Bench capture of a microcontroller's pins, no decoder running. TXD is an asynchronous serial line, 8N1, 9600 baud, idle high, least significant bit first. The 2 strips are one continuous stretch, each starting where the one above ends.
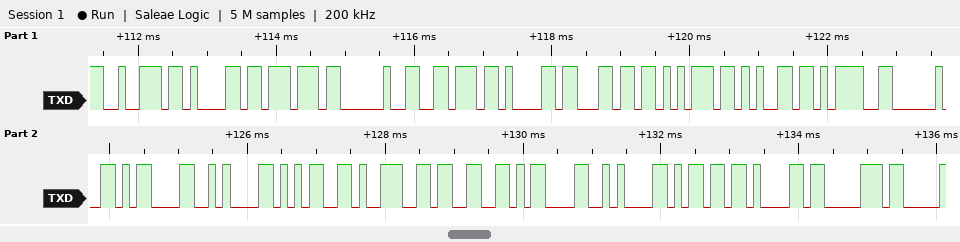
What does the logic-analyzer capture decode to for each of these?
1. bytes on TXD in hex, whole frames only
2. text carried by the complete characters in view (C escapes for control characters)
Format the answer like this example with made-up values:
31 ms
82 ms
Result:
72 61 77 20 76 61 6C 75 65 3D 20 0D 0A 35 39 33 0D 0A 6D 61 70
"raw value= \r\n593\r\nmap"
